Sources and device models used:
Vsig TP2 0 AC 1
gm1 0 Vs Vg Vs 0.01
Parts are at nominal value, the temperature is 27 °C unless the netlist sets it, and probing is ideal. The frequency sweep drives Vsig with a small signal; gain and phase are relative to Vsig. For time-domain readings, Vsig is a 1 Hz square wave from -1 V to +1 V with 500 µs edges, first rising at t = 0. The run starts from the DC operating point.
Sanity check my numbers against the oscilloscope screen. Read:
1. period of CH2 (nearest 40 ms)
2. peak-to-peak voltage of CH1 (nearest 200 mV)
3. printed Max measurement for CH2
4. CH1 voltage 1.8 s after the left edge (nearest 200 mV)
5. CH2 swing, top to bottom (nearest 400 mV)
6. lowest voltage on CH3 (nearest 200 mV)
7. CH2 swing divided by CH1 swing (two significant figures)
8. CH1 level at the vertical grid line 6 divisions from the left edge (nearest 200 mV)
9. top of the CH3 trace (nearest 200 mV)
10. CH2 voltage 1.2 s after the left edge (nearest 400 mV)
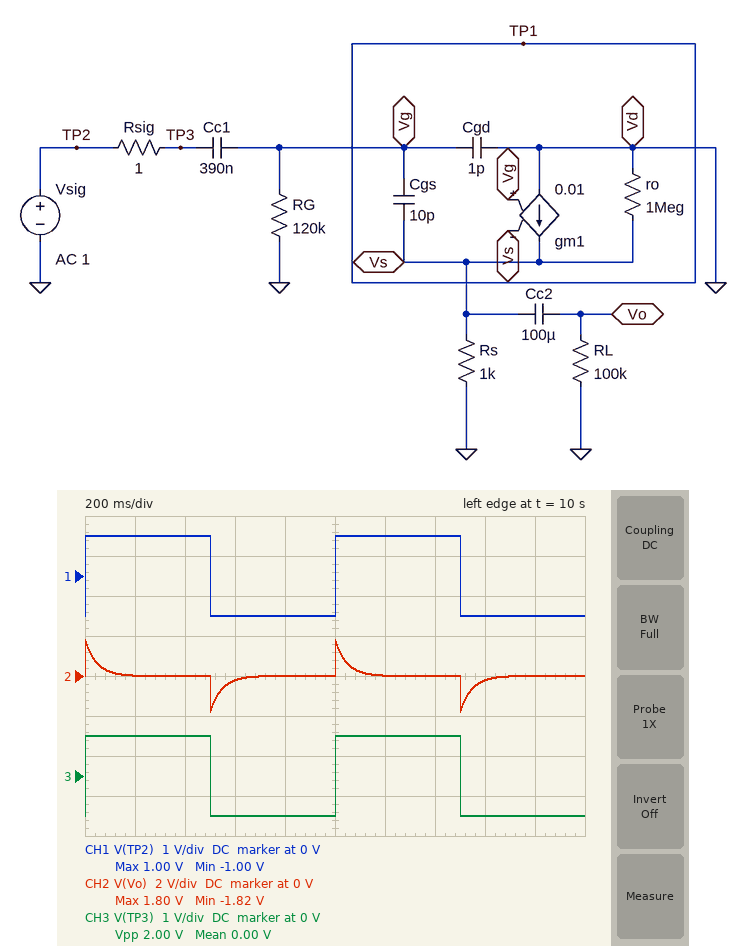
1.00 s
2.0 V
1.80 V
-1.0 V
3.6 V
-1.0 V
1.8
1.0 V
1.0 V
0 V
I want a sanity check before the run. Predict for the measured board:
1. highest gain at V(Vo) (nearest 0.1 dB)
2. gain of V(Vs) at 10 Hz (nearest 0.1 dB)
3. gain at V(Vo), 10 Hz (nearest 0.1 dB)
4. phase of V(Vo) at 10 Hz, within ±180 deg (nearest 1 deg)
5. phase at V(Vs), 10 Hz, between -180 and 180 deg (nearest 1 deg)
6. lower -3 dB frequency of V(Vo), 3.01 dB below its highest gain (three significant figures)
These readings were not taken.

-0.8 dB
-1.3 dB
-1.3 dB
19 deg
19 deg
3.40 Hz
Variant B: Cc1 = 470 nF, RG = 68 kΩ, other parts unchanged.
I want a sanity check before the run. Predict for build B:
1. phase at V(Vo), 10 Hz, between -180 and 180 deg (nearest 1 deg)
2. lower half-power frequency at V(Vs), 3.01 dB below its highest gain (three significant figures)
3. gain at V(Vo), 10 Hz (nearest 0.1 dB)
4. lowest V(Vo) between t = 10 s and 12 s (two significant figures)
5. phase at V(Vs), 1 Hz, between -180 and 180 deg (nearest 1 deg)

27 deg
4.98 Hz
-1.8 dB
-1.8 V
79 deg
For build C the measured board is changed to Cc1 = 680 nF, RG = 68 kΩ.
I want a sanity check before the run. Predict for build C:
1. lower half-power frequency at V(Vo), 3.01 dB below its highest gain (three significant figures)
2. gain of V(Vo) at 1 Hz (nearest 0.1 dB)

3.44 Hz
-11.9 dB
